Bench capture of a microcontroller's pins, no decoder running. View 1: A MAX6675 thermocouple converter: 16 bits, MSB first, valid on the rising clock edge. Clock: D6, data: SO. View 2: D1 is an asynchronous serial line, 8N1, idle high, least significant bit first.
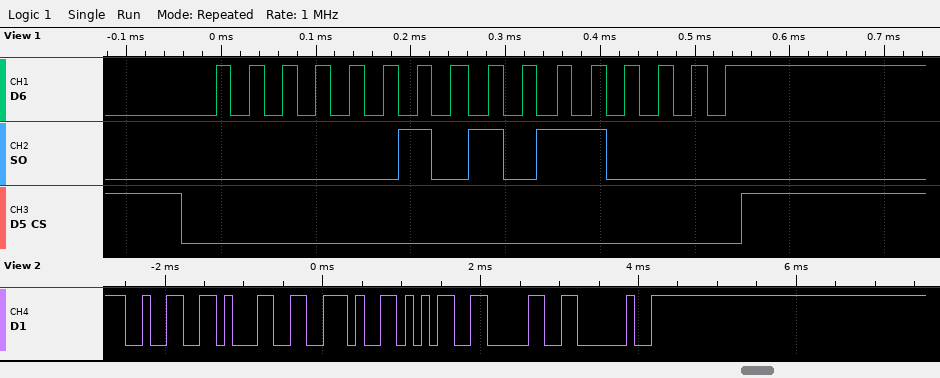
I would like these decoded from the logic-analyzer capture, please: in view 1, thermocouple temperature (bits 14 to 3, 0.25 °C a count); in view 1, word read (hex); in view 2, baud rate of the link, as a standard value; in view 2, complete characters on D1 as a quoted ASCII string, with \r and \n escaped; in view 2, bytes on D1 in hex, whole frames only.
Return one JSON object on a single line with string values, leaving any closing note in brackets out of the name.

{"in view 1, thermocouple temperature": "21.50 °C", "in view 1, word read": "0x02B0", "in view 2, baud rate of the link, as a standard value": "9600 baud", "in view 2, complete characters on D1 as a quoted ASCII string, with \\r and \\n escaped": "\"21.50 \"", "in view 2, bytes on D1 in hex, whole frames only": "32 31 2E 35 30 20"}
